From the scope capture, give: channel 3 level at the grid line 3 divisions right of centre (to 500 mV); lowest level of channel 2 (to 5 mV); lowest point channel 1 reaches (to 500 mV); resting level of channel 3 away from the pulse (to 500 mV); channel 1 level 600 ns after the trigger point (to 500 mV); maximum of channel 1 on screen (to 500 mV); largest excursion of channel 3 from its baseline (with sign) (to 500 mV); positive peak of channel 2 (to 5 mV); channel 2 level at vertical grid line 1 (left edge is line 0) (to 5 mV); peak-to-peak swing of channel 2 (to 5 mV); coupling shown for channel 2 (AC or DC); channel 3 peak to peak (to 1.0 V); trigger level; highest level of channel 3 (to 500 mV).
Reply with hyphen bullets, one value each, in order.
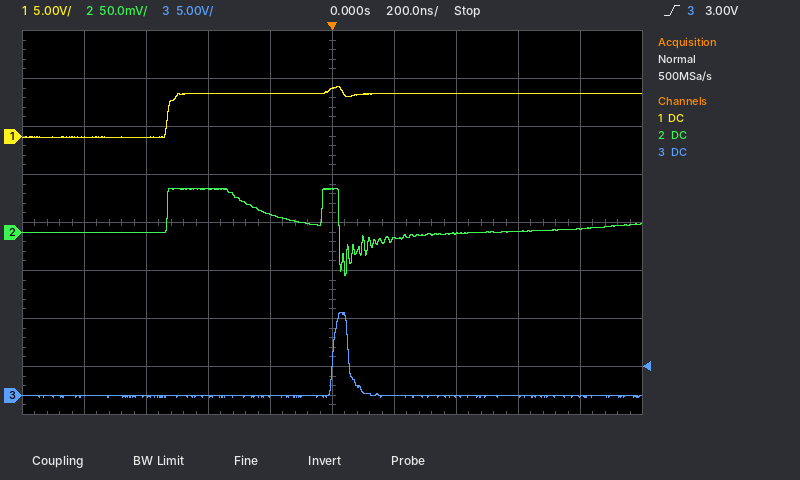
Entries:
- 0.0 V
- -45 mV
- 0.0 V
- 0.0 V
- 4.5 V
- 5.0 V
- +8.5 V
- 45 mV
- 0 mV
- 90 mV
- DC
- 9.0 V
- 3.00 V
- 8.5 V
